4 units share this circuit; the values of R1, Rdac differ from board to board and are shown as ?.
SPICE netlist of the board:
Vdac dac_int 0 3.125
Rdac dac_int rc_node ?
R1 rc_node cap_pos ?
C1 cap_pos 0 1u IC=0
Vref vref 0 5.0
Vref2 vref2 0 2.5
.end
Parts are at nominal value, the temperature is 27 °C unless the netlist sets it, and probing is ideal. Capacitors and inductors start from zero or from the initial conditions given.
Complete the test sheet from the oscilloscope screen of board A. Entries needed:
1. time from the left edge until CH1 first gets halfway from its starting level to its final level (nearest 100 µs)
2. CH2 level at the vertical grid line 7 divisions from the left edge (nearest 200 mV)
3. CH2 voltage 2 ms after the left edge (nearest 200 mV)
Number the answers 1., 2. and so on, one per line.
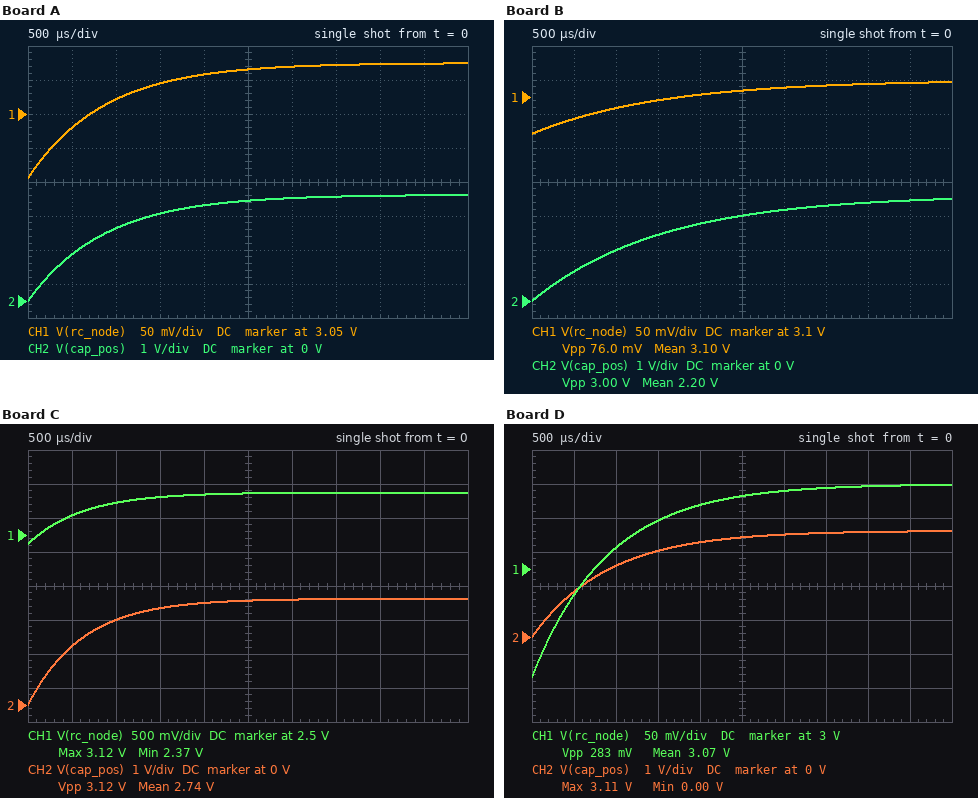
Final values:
1. 600 µs
2. 3.0 V
3. 2.8 V
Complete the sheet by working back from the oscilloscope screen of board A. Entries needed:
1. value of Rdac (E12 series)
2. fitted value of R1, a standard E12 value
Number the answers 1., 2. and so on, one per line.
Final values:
1. 47 Ω
2. 820 Ω
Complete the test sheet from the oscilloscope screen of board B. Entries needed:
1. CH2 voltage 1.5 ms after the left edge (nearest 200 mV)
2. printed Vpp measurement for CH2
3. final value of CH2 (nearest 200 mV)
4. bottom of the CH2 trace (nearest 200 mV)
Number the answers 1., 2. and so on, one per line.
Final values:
1. 2.0 V
2. 3.00 V
3. 3.0 V
4. 0 V
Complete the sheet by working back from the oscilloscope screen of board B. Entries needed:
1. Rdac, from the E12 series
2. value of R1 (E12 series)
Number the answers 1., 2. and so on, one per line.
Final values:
1. 39 Ω
2. 1.5 kΩ
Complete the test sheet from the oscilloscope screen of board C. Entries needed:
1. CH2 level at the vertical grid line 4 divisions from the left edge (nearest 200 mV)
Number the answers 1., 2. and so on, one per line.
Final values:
1. 3.0 V
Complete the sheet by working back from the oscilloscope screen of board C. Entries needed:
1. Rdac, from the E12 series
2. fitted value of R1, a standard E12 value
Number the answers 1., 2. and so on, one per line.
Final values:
1. 150 Ω
2. 470 Ω
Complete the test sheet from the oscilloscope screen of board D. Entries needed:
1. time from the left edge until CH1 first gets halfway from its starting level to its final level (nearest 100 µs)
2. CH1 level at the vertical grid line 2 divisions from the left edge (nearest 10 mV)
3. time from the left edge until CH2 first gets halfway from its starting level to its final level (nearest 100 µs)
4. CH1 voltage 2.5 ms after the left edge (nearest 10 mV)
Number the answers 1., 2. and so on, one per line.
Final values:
1. 600 µs
2. 3.03 V
3. 600 µs
4. 3.11 V
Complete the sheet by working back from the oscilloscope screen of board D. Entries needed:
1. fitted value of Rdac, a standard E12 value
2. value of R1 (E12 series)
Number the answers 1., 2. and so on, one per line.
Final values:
1. 82 Ω
2. 820 Ω
